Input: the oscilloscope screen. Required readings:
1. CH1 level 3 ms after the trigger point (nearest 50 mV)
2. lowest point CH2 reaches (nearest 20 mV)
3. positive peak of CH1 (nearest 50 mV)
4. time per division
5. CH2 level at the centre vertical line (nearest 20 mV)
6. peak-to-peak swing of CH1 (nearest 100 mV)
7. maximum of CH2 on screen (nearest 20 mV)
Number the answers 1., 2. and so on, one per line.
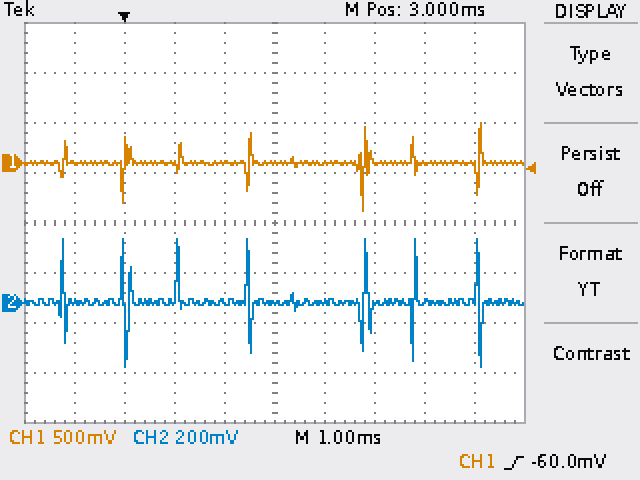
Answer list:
1. 0 mV
2. -260 mV
3. 400 mV
4. 1 ms
5. 0 mV
6. 900 mV
7. 260 mV
